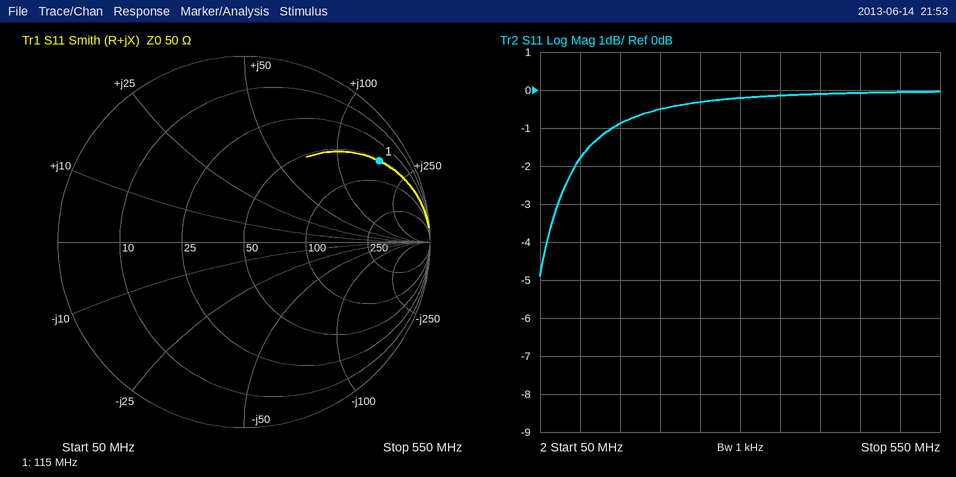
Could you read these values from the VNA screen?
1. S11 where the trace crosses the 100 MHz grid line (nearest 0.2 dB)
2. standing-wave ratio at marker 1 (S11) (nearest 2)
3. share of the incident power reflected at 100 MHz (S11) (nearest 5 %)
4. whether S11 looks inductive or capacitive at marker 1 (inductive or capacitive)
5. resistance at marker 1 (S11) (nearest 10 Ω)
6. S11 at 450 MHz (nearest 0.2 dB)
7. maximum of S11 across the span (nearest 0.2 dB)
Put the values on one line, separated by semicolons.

-1.8 dB; 12; 65 %; inductive; 50 Ω; 0.0 dB; 0.0 dB
